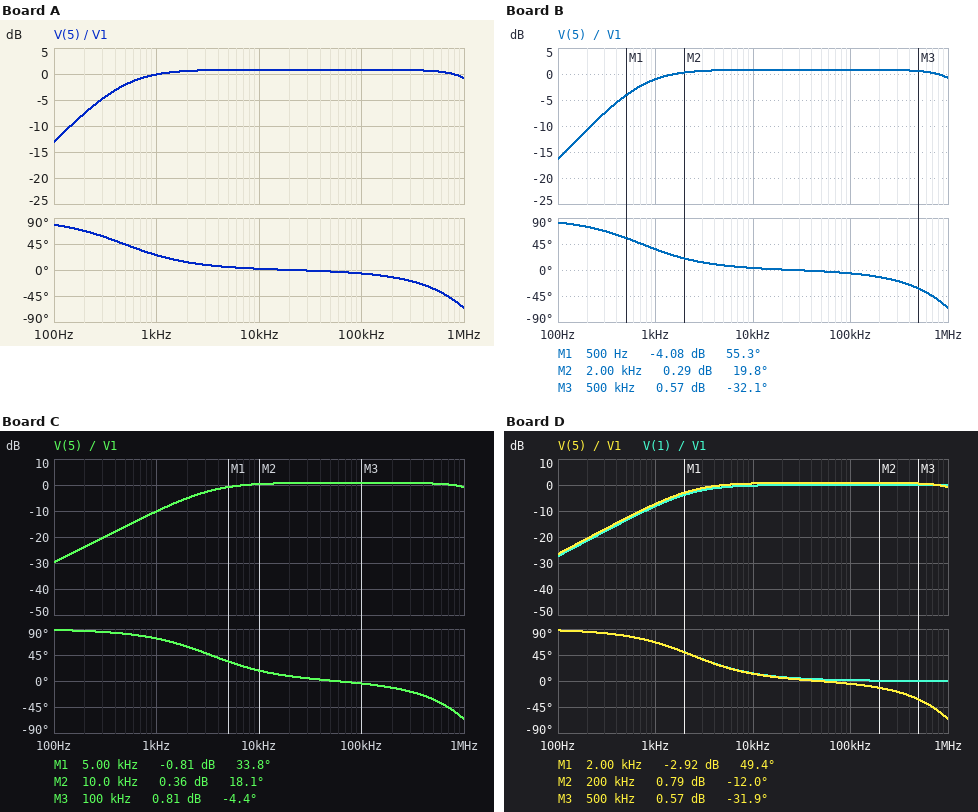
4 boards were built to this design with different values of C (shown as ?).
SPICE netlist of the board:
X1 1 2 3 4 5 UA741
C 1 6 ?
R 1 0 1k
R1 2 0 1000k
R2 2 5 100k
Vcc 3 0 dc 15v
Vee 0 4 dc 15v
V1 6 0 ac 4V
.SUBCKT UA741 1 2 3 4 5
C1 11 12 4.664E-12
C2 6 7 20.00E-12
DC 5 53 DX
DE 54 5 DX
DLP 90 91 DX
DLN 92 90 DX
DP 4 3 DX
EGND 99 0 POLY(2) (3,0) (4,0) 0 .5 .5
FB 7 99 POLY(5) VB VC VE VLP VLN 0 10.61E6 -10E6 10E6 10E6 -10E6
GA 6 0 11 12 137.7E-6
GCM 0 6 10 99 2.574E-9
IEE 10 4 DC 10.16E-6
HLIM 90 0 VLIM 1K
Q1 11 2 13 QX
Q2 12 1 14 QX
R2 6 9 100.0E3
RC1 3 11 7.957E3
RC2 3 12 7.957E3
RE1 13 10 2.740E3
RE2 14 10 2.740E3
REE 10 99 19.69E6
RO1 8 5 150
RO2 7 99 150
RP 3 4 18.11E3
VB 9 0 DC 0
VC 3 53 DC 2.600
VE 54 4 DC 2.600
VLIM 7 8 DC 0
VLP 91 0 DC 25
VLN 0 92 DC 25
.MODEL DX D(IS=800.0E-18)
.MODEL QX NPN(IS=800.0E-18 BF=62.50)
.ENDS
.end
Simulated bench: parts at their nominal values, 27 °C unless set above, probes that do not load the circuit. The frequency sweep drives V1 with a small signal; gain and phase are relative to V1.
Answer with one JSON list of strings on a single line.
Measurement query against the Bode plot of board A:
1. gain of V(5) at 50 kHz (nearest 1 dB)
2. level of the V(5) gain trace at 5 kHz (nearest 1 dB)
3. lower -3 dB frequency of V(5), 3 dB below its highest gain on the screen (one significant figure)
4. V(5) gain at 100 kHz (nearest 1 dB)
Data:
["1 dB", "1 dB", "500 Hz", "1 dB"]
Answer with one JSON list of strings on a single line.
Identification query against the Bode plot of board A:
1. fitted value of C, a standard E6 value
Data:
["330 nF"]
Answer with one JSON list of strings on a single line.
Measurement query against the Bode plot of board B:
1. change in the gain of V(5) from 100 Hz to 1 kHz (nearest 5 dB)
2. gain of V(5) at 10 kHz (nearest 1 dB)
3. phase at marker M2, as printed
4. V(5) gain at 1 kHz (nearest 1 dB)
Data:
["15 dB", "1 dB", "19.8 deg", "-1 dB"]
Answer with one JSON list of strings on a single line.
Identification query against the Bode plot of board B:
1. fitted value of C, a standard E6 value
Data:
["220 nF"]
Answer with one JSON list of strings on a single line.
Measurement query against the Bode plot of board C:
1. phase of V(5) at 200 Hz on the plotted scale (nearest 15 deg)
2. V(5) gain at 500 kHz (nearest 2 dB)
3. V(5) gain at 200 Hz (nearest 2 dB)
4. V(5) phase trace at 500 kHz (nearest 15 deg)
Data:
["90 deg", "0 dB", "-24 dB", "-30 deg"]
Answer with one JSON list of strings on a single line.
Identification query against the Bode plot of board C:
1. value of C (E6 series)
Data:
["47 nF"]
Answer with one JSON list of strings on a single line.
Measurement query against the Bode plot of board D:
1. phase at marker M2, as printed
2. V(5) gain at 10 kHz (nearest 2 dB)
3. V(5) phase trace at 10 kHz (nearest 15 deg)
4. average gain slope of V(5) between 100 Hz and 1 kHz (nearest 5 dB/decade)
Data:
["-12.0 deg", "0 dB", "15 deg", "20 dB/decade"]
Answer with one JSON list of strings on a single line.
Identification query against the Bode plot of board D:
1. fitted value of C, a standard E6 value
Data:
["68 nF"]
